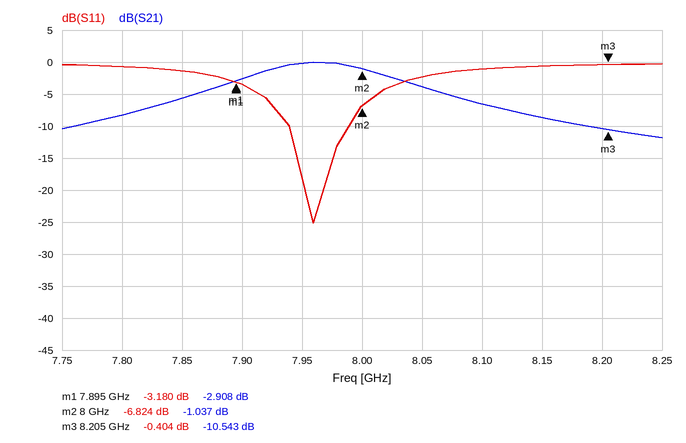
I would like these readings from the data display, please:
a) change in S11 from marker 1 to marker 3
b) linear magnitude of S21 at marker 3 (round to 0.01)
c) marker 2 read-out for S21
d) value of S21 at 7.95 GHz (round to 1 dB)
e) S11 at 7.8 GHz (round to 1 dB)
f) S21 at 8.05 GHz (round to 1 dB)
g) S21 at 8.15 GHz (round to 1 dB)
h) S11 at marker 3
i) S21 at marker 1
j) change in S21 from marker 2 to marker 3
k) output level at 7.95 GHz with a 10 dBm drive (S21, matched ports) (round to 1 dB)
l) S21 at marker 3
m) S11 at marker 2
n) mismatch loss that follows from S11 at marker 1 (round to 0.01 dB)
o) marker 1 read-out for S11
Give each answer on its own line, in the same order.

2.776 dB
0.30
-1.037 dB
0 dB
-1 dB
-4 dB
-9 dB
-0.404 dB
-2.908 dB
-9.506 dB
10 dBm
-10.543 dB
-6.824 dB
2.85 dB
-3.180 dB
